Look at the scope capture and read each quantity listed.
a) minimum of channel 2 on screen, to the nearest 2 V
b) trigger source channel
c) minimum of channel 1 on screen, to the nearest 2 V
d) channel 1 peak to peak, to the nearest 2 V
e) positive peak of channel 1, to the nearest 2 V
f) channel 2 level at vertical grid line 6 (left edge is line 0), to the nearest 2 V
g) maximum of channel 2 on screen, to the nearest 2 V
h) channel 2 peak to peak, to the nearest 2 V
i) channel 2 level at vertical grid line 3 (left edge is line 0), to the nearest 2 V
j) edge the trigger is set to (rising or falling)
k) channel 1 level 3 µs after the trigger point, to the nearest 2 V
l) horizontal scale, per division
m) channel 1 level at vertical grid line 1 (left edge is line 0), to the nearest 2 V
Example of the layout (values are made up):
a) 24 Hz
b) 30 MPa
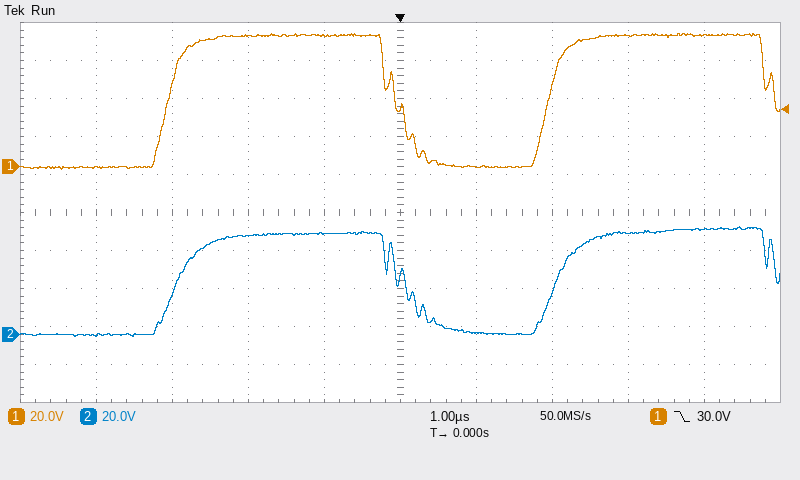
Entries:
a) -2 V
b) channel 1
c) -2 V
d) 72 V
e) 70 V
f) 0 V
g) 56 V
h) 58 V
i) 52 V
j) falling
k) 70 V
l) 1 µs
m) 0 V
